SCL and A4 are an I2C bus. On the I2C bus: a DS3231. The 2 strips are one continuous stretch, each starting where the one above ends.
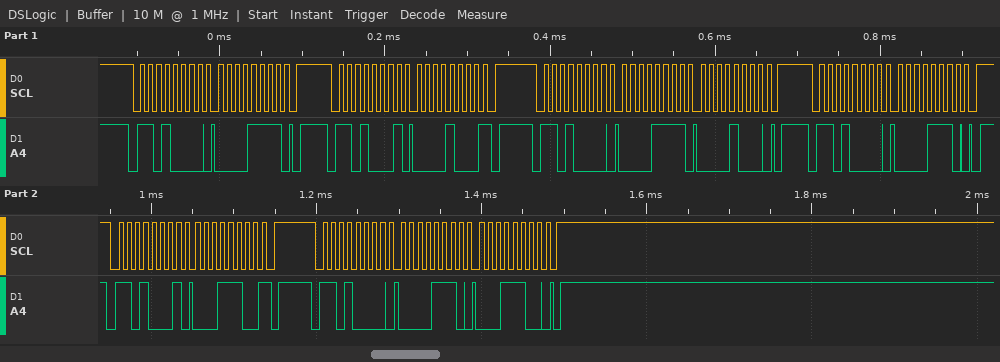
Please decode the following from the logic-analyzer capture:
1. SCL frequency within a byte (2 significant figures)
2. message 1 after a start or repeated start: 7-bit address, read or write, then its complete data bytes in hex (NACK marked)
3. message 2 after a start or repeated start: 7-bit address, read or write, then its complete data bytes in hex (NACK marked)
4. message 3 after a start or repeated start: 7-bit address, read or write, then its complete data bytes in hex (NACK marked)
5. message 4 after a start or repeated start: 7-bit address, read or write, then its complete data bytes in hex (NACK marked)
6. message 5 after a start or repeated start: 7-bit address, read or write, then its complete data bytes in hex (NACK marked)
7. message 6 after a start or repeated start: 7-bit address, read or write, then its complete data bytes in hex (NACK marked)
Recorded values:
100 kHz
0x68 write: 0F
0x68 read: 08 NACK
0x68 write: 0F 08
0x68 write: 0E
0x68 read: 1C NACK
0x68 write: 0E 1C
